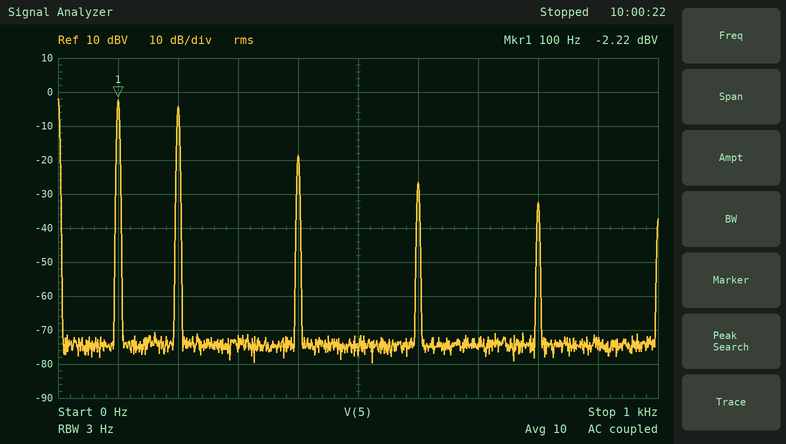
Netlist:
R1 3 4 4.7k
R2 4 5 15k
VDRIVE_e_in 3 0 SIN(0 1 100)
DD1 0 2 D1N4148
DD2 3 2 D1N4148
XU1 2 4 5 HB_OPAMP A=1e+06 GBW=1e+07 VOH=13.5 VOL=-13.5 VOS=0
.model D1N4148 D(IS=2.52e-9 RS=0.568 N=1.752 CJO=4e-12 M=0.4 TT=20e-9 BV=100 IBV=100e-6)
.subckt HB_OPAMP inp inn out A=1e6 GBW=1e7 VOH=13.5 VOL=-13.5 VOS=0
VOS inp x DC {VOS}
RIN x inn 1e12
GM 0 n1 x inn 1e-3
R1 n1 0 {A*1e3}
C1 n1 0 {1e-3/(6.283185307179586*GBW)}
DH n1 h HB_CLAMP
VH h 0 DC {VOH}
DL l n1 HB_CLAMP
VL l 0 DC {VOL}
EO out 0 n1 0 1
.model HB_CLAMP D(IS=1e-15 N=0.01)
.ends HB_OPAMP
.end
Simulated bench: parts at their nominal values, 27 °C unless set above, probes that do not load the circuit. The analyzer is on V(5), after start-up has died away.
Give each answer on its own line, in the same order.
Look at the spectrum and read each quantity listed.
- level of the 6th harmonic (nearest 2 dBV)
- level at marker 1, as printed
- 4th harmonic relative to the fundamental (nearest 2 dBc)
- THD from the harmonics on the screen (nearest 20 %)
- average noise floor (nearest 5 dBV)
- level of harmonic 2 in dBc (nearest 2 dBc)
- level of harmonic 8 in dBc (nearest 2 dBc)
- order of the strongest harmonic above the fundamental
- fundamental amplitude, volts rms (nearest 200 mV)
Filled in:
-26 dBV
-2.22 dBV
-16 dBc
80 %
-75 dBV
-2 dBc
-30 dBc
2
800 mV
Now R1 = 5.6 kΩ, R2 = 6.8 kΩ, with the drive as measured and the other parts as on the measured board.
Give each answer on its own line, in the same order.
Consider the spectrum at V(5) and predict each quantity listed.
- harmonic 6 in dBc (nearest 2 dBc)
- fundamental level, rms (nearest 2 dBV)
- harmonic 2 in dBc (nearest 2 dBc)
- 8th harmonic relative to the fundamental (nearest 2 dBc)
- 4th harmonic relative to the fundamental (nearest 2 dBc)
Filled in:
-10 dBc
-22 dBV
12 dBc
-16 dBc
-2 dBc
